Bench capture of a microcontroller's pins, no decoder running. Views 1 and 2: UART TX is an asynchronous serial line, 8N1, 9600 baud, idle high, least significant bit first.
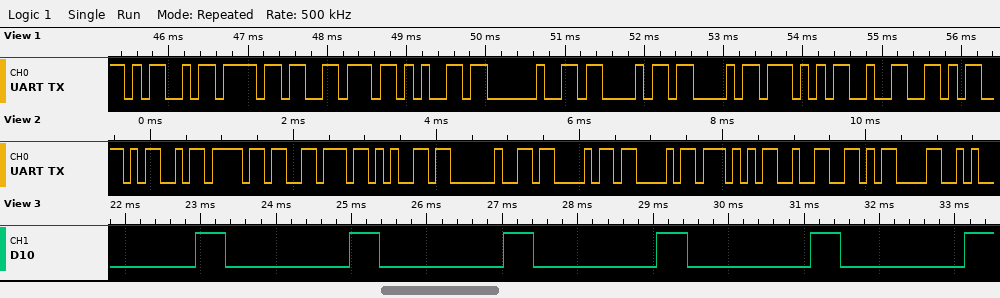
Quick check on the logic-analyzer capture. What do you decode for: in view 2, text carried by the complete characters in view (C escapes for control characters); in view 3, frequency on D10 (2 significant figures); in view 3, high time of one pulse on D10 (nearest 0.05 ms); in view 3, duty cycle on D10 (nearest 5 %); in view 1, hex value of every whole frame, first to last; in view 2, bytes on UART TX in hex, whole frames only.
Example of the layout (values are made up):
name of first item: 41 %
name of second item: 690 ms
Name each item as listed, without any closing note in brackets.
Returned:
in view 2, text carried by the complete characters in view: "Move CCW2\r"
in view 3, frequency on D10: 490 Hz
in view 3, high time of one pulse on D10: 0.40 ms
in view 3, duty cycle on D10: 20 %
in view 1, hex value of every whole frame, first to last: 4D 6F 76 65 20 43 43 57 32
in view 2, bytes on UART TX in hex, whole frames only: 4D 6F 76 65 20 43 43 57 32 0D
